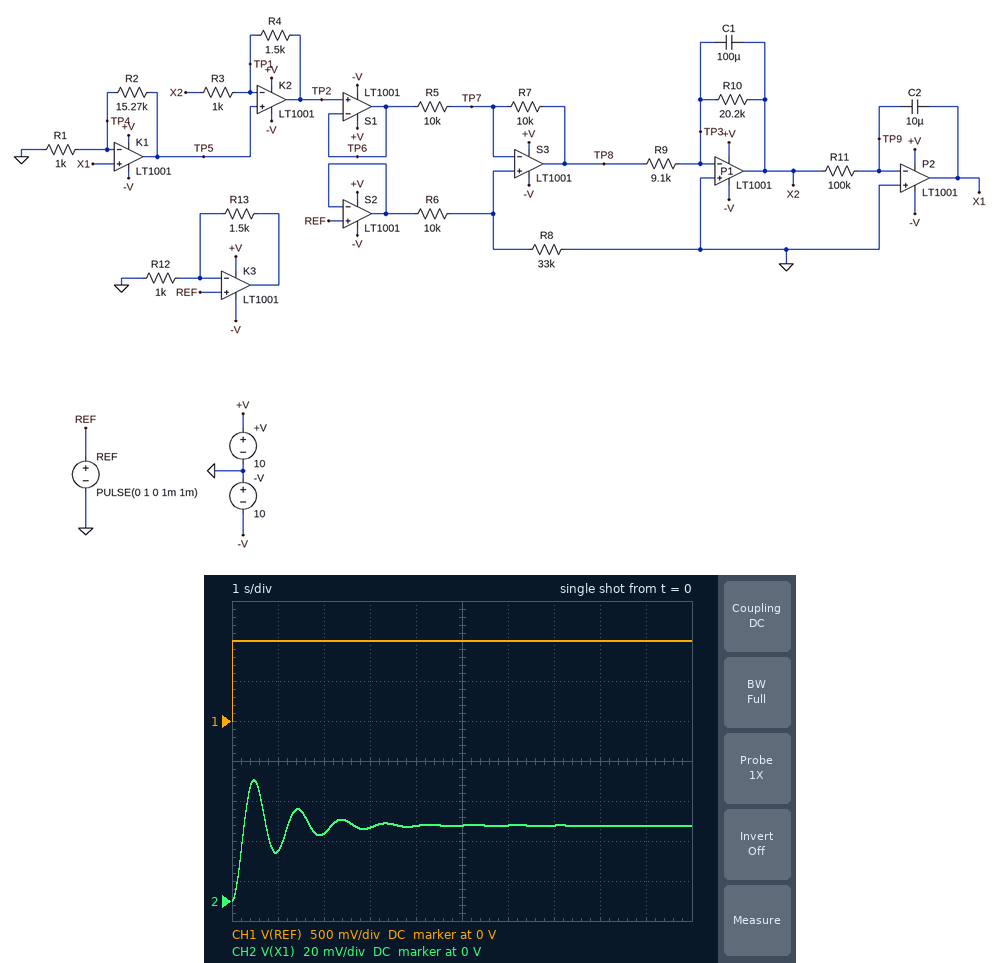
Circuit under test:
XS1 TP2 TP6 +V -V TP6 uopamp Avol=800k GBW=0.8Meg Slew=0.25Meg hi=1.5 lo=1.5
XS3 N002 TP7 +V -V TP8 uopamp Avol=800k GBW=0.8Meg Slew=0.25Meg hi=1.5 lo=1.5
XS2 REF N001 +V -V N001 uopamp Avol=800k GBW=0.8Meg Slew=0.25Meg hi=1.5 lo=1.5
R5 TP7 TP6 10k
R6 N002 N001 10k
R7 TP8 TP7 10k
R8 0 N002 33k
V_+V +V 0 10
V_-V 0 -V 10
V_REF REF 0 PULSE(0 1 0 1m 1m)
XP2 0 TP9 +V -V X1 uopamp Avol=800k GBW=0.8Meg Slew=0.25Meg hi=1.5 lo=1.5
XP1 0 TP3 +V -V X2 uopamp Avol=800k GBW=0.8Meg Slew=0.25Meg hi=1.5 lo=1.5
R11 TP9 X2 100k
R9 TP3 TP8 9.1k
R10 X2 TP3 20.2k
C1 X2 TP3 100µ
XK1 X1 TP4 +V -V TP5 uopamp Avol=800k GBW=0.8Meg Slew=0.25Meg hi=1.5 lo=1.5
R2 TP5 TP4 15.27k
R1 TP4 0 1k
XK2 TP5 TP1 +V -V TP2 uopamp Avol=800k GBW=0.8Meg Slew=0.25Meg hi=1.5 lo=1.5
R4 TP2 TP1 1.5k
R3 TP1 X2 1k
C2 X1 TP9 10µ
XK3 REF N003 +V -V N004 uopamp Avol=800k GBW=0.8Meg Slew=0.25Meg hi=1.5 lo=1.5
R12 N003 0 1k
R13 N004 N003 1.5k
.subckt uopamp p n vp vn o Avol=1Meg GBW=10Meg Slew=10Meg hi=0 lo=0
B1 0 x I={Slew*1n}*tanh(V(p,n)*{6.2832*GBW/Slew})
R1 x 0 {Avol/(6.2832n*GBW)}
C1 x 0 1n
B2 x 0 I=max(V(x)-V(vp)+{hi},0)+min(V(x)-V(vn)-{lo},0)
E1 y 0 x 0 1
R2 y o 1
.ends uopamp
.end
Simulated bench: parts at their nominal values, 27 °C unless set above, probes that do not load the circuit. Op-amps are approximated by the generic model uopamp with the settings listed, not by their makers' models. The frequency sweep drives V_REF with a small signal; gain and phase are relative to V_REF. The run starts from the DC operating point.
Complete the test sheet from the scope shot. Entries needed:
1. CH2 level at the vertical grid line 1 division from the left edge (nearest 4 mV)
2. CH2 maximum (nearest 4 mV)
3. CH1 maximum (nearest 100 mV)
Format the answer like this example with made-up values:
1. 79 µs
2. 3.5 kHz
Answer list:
1. 24 mV
2. 60 mV
3. 1.0 V
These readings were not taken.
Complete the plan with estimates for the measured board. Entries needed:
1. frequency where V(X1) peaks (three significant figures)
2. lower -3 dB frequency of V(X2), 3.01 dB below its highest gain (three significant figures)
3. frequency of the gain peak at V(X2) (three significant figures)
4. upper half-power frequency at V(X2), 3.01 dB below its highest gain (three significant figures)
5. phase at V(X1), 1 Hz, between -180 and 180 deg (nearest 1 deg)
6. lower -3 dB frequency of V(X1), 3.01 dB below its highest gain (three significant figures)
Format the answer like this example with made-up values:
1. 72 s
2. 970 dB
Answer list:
1. 1.04 Hz
2. 907 mHz
3. 1.06 Hz
4. 1.25 Hz
5. -69 deg
6. 846 mHz
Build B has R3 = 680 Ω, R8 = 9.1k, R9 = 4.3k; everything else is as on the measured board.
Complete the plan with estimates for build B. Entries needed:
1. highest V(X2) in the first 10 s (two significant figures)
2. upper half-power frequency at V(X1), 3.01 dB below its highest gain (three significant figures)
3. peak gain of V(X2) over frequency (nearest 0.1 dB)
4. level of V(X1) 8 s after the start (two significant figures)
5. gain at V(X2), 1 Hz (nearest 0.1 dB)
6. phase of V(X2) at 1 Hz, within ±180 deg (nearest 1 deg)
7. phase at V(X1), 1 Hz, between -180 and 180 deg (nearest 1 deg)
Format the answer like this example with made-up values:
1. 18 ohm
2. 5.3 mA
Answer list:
1. 62 mV
2. 2.05 Hz
3. -8.1 dB
4. 18 mV
5. -16.1 dB
6. -113 deg
7. -23 deg
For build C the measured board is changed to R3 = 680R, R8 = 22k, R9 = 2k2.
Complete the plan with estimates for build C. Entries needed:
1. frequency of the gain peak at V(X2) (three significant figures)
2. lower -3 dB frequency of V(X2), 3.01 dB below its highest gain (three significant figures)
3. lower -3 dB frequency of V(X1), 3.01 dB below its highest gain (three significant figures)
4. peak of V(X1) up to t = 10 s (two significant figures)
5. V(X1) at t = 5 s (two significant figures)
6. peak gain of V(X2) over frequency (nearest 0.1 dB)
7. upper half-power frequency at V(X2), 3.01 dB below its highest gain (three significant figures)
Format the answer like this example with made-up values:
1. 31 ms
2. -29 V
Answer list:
1. 2.45 Hz
2. 1.75 Hz
3. 864 mHz
4. 35 mV
5. 26 mV
6. -4.5 dB
7. 3.43 Hz
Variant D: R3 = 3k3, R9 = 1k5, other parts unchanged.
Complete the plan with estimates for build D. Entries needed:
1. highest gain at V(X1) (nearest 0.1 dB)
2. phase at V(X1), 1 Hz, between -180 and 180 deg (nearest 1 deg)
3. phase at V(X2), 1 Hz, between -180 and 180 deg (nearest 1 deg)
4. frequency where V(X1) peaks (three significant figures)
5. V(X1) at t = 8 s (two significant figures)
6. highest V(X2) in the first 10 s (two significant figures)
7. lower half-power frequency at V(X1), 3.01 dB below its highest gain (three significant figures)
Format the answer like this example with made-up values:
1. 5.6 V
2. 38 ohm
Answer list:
1. -12.6 dB
2. -11 deg
3. -101 deg
4. 1.96 Hz
5. 65 mV
6. 430 mV
7. 1.65 Hz
